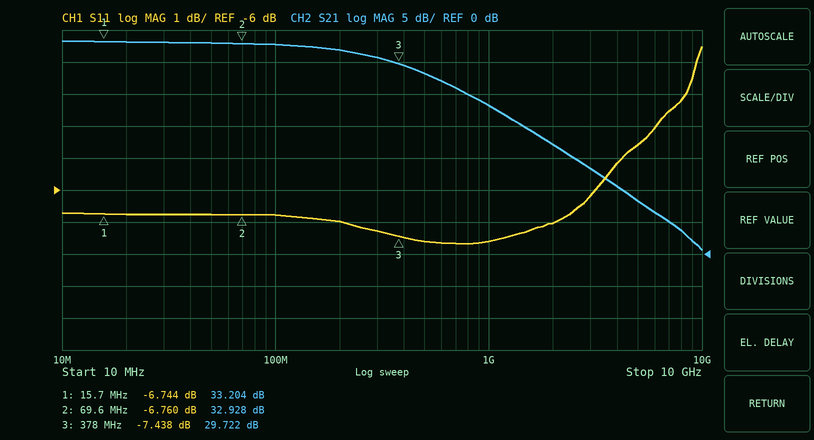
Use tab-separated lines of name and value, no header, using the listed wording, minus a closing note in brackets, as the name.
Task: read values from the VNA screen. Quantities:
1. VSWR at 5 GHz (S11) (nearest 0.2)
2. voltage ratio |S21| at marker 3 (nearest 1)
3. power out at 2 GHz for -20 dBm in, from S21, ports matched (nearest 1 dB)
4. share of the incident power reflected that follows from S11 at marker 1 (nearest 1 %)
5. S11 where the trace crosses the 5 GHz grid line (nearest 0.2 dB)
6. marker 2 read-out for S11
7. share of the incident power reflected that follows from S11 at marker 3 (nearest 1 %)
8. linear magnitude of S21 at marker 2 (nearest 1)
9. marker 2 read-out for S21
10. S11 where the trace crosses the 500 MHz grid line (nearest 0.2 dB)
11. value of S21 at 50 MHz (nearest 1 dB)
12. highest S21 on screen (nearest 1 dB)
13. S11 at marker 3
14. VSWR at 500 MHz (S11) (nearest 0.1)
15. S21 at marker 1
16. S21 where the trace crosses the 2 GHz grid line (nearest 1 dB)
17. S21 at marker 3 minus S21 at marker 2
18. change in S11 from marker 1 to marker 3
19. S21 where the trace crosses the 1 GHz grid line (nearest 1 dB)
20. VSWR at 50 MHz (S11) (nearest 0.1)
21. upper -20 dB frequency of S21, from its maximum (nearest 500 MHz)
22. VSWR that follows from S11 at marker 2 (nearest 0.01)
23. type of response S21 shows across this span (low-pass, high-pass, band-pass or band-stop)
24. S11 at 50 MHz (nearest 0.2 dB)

VSWR at 5 GHz (S11)	3.8
voltage ratio |S21| at marker 3	31
power out at 2 GHz for -20 dBm in, from S21, ports matched	-3 dBm
share of the incident power reflected that follows from S11 at marker 1	21 %
S11 where the trace crosses the 5 GHz grid line	-4.6 dB
marker 2 read-out for S11	-6.760 dB
share of the incident power reflected that follows from S11 at marker 3	18 %
linear magnitude of S21 at marker 2	44
marker 2 read-out for S21	32.928 dB
S11 where the trace crosses the 500 MHz grid line	-7.6 dB
value of S21 at 50 MHz	33 dB
highest S21 on screen	33 dB
S11 at marker 3	-7.438 dB
VSWR at 500 MHz (S11)	2.4
S21 at marker 1	33.204 dB
S21 where the trace crosses the 2 GHz grid line	17 dB
S21 at marker 3 minus S21 at marker 2	-3.206 dB
change in S11 from marker 1 to marker 3	-0.694 dB
S21 where the trace crosses the 1 GHz grid line	23 dB
VSWR at 50 MHz (S11)	2.7
upper -20 dB frequency of S21, from its maximum	3.0 GHz
VSWR that follows from S11 at marker 2	2.70
type of response S21 shows across this span	low-pass
S11 at 50 MHz	-6.8 dB
